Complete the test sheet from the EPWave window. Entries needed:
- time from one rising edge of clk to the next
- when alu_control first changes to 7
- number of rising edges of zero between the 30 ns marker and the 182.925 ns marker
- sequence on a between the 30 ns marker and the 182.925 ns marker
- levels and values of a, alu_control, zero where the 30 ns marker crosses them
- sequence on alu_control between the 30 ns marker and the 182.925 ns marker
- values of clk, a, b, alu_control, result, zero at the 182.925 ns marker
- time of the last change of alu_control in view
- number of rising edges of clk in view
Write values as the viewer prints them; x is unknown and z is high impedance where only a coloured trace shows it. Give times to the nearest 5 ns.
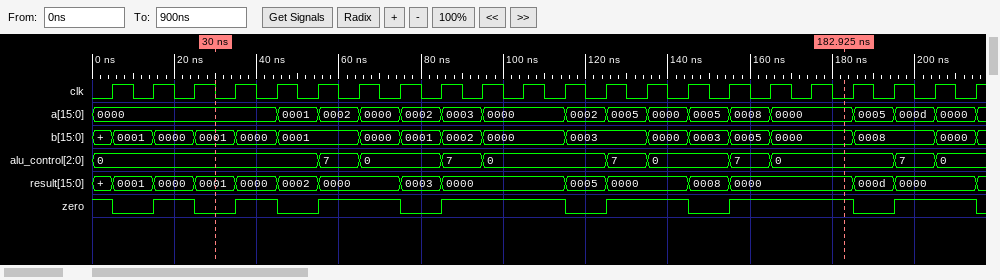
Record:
10 ns
55 ns
5
0000, 0001, 0002, 0000, 0002, 0003, 0000, 0002, 0005, 0000, 0005, 0008, 0000
a=0000, alu_control=0, zero=0
0, 7, 0, 7, 0, 7, 0, 7, 0
clk=0, a=0000, b=0000, alu_control=0, result=0000, zero=1
205 ns
22
